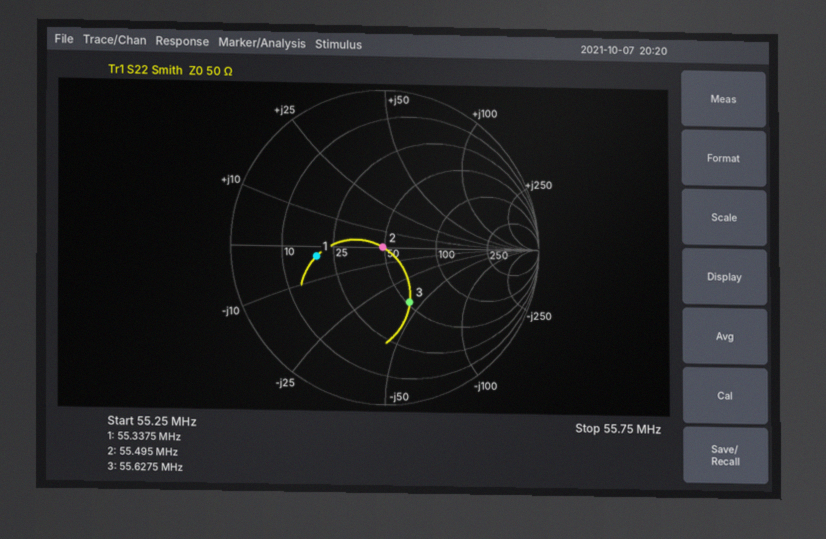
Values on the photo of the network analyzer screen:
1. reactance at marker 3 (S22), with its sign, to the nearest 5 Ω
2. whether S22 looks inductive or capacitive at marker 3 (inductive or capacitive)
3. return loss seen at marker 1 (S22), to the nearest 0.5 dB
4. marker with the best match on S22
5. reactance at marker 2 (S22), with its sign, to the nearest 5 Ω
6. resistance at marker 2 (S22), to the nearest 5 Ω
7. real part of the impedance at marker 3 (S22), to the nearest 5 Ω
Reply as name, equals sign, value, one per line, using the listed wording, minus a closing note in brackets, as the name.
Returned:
reactance at marker 3 (S22), with its sign, to the nearest 5 Ω = -40 Ω
whether S22 looks inductive or capacitive at marker 3 = capacitive
return loss seen at marker 1 (S22), to the nearest 0.5 dB = 7.0 dB
marker with the best match on S22 = marker 2
reactance at marker 2 (S22), with its sign, to the nearest 5 Ω = 0 Ω
resistance at marker 2 (S22), to the nearest 5 Ω = 50 Ω
real part of the impedance at marker 3 (S22), to the nearest 5 Ω = 50 Ω
